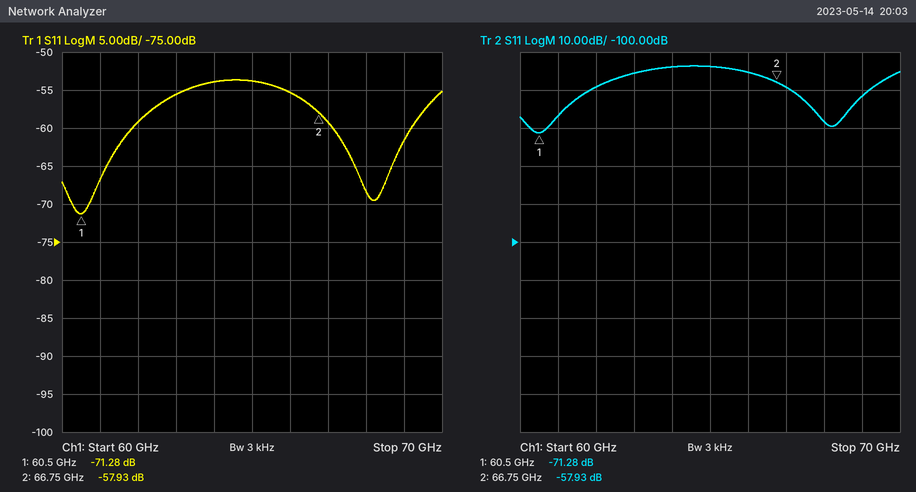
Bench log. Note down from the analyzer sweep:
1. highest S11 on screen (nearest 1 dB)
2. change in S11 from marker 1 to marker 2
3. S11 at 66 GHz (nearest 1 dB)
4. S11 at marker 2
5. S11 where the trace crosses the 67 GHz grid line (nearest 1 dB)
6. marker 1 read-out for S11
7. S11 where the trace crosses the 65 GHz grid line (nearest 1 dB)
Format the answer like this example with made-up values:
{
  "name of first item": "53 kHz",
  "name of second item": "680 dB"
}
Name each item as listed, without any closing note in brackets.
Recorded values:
{
  "highest S11 on screen": "-54 dB",
  "change in S11 from marker 1 to marker 2": "13.35 dB",
  "S11 at 66 GHz": "-55 dB",
  "S11 at marker 2": "-57.93 dB",
  "S11 where the trace crosses the 67 GHz grid line": "-59 dB",
  "marker 1 read-out for S11": "-71.28 dB",
  "S11 where the trace crosses the 65 GHz grid line": "-54 dB"
}
